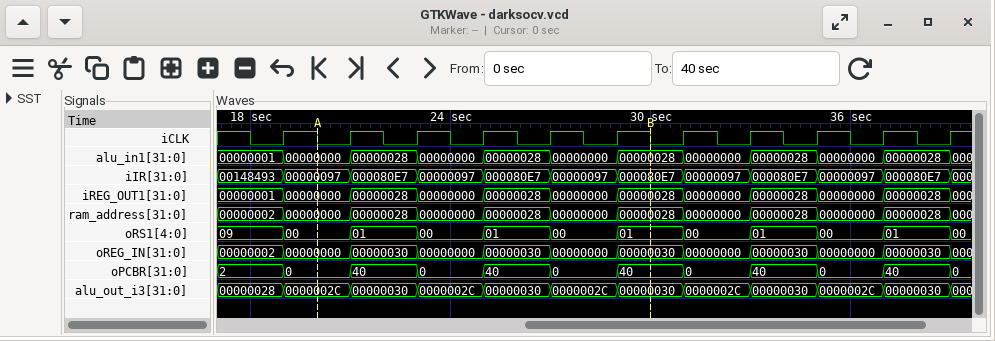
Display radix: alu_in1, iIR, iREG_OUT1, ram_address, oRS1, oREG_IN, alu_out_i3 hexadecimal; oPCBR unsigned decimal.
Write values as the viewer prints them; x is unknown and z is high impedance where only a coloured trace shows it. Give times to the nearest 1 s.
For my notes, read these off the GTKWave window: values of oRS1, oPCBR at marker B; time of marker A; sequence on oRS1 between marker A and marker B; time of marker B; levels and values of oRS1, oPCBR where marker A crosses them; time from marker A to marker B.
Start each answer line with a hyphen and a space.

- oRS1=01, oPCBR=40
- 20 s
- 00, 01, 00, 01, 00, 01
- 30 s
- oRS1=00, oPCBR=0
- 10 s
